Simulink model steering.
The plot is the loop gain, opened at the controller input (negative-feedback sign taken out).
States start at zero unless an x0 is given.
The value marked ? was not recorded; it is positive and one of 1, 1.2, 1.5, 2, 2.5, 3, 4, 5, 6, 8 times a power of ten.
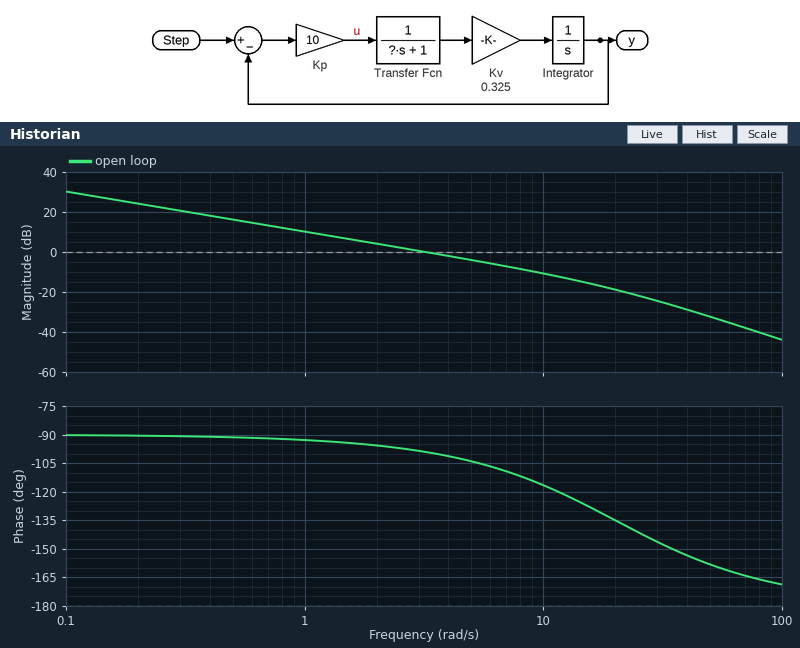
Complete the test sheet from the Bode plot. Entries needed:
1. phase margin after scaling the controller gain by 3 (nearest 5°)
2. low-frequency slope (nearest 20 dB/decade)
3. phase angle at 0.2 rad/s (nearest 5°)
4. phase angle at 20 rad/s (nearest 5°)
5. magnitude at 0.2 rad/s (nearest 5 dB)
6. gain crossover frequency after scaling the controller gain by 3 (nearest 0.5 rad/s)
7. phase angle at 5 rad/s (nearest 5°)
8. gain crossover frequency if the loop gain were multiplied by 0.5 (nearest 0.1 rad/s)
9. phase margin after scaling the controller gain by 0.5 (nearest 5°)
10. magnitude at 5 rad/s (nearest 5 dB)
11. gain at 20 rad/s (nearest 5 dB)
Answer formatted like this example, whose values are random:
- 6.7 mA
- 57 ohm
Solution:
- 65°
- -20 dB/decade
- -90°
- -135°
- 25 dB
- 9.0 rad/s
- -105°
- 1.6 rad/s
- 85°
- -5 dB
- -20 dB
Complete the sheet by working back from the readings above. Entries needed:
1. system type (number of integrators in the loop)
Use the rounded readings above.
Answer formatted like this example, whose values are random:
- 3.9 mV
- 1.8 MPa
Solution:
- 1
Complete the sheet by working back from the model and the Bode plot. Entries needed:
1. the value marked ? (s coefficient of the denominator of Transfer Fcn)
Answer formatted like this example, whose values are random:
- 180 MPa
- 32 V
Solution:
- 0.05
